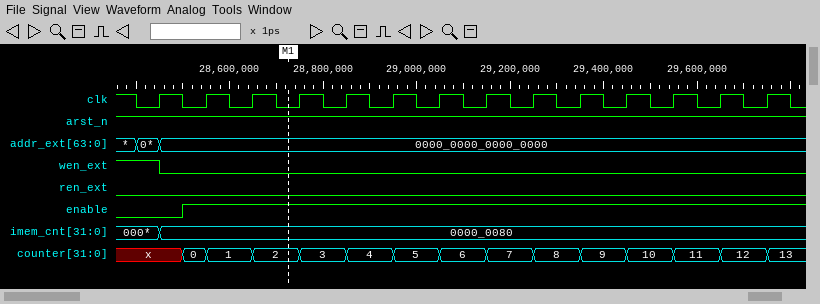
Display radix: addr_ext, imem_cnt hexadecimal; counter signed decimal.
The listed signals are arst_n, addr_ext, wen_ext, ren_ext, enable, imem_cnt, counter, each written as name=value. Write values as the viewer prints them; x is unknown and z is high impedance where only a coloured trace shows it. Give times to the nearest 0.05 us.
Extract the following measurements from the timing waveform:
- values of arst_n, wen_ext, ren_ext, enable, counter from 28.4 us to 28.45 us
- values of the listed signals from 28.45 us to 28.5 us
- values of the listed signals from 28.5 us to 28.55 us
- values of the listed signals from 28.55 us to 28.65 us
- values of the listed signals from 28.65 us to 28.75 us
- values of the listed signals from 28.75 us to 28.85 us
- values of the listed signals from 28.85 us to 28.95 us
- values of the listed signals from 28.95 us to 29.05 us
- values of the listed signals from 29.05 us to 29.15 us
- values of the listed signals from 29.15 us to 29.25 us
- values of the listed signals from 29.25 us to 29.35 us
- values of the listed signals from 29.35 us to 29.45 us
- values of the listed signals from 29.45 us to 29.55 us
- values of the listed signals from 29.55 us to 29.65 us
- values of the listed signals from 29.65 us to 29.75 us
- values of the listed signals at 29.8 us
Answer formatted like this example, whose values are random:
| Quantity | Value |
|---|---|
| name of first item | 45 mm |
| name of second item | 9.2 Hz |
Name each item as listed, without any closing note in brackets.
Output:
| Quantity | Value |
|---|---|
| values of arst_n, wen_ext, ren_ext, enable, counter from 28.4 us to 28.45 us | arst_n=1, wen_ext=1, ren_ext=0, enable=0, counter=x |
| values of the listed signals from 28.45 us to 28.5 us | arst_n=1, addr_ext=0000_0000_0000_0000, wen_ext=0, ren_ext=0, enable=0, imem_cnt=0000_0080, counter=x |
| values of the listed signals from 28.5 us to 28.55 us | arst_n=1, addr_ext=0000_0000_0000_0000, wen_ext=0, ren_ext=0, enable=1, imem_cnt=0000_0080, counter=0 |
| values of the listed signals from 28.55 us to 28.65 us | arst_n=1, addr_ext=0000_0000_0000_0000, wen_ext=0, ren_ext=0, enable=1, imem_cnt=0000_0080, counter=1 |
| values of the listed signals from 28.65 us to 28.75 us | arst_n=1, addr_ext=0000_0000_0000_0000, wen_ext=0, ren_ext=0, enable=1, imem_cnt=0000_0080, counter=2 |
| values of the listed signals from 28.75 us to 28.85 us | arst_n=1, addr_ext=0000_0000_0000_0000, wen_ext=0, ren_ext=0, enable=1, imem_cnt=0000_0080, counter=3 |
| values of the listed signals from 28.85 us to 28.95 us | arst_n=1, addr_ext=0000_0000_0000_0000, wen_ext=0, ren_ext=0, enable=1, imem_cnt=0000_0080, counter=4 |
| values of the listed signals from 28.95 us to 29.05 us | arst_n=1, addr_ext=0000_0000_0000_0000, wen_ext=0, ren_ext=0, enable=1, imem_cnt=0000_0080, counter=5 |
| values of the listed signals from 29.05 us to 29.15 us | arst_n=1, addr_ext=0000_0000_0000_0000, wen_ext=0, ren_ext=0, enable=1, imem_cnt=0000_0080, counter=6 |
| values of the listed signals from 29.15 us to 29.25 us | arst_n=1, addr_ext=0000_0000_0000_0000, wen_ext=0, ren_ext=0, enable=1, imem_cnt=0000_0080, counter=7 |
| values of the listed signals from 29.25 us to 29.35 us | arst_n=1, addr_ext=0000_0000_0000_0000, wen_ext=0, ren_ext=0, enable=1, imem_cnt=0000_0080, counter=8 |
| values of the listed signals from 29.35 us to 29.45 us | arst_n=1, addr_ext=0000_0000_0000_0000, wen_ext=0, ren_ext=0, enable=1, imem_cnt=0000_0080, counter=9 |
| values of the listed signals from 29.45 us to 29.55 us | arst_n=1, addr_ext=0000_0000_0000_0000, wen_ext=0, ren_ext=0, enable=1, imem_cnt=0000_0080, counter=10 |
| values of the listed signals from 29.55 us to 29.65 us | arst_n=1, addr_ext=0000_0000_0000_0000, wen_ext=0, ren_ext=0, enable=1, imem_cnt=0000_0080, counter=11 |
| values of the listed signals from 29.65 us to 29.75 us | arst_n=1, addr_ext=0000_0000_0000_0000, wen_ext=0, ren_ext=0, enable=1, imem_cnt=0000_0080, counter=12 |
| values of the listed signals at 29.8 us | arst_n=1, addr_ext=0000_0000_0000_0000, wen_ext=0, ren_ext=0, enable=1, imem_cnt=0000_0080, counter=13 |
